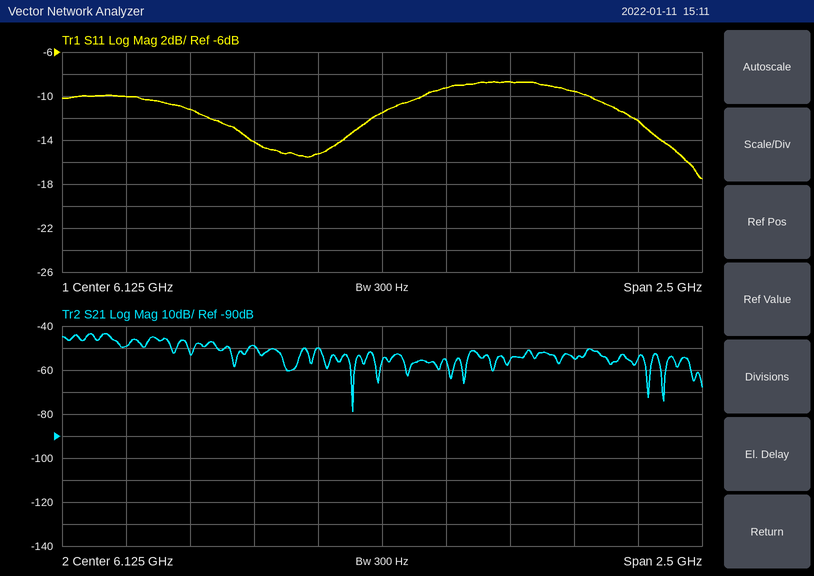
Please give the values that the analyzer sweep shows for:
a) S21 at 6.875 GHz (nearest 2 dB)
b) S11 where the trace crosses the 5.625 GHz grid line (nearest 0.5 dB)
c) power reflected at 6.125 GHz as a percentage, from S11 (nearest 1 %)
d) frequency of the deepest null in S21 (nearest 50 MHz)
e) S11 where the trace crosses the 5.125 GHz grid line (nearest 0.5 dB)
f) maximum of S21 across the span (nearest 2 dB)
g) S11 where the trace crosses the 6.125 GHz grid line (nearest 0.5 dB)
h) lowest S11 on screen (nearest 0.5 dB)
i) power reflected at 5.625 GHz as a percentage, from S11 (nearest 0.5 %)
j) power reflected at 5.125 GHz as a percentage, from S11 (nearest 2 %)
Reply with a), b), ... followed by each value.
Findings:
a) -54 dB
b) -14.0 dB
c) 7 %
d) 6.00 GHz
e) -10.0 dB
f) -44 dB
g) -11.5 dB
h) -17.5 dB
i) 4.0 %
j) 10 %
